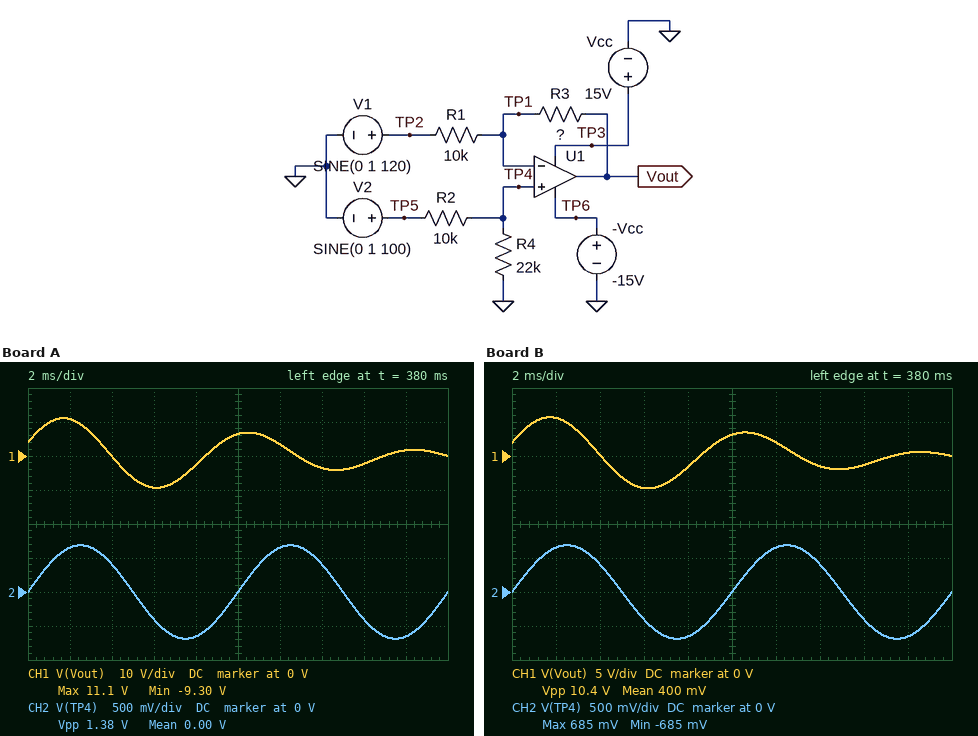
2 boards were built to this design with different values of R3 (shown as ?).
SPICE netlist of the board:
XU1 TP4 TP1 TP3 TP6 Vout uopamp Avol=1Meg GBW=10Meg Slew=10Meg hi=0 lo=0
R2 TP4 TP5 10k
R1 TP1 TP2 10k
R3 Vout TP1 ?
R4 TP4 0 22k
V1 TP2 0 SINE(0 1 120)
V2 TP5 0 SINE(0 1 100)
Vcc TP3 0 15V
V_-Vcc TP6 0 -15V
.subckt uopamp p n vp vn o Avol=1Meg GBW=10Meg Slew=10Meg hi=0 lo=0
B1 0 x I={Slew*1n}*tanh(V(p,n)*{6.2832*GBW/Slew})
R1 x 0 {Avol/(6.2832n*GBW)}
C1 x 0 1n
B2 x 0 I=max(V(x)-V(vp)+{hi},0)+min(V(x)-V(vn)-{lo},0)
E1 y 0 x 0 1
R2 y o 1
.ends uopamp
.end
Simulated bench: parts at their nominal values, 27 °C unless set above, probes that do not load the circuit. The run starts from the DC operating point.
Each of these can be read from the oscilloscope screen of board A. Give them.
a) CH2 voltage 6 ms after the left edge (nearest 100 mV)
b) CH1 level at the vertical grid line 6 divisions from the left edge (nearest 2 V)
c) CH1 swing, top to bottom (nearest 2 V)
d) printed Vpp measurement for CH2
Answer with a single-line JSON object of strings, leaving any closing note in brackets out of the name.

{"CH2 voltage 6 ms after the left edge": "-400 mV", "CH1 level at the vertical grid line 6 divisions from the left edge": "4 V", "CH1 swing, top to bottom": "20 V", "printed Vpp measurement for CH2": "1.38 V"}
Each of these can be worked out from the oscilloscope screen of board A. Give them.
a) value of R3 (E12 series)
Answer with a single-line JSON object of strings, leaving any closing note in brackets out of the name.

{"value of R3": "68 kΩ"}
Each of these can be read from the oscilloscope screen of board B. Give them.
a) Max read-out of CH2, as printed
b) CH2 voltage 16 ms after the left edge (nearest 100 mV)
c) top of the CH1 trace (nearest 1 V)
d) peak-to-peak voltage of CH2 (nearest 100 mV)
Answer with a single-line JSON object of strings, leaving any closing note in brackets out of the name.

{"Max read-out of CH2, as printed": "685 mV", "CH2 voltage 16 ms after the left edge": "-400 mV", "top of the CH1 trace": "6 V", "peak-to-peak voltage of CH2": "1.4 V"}
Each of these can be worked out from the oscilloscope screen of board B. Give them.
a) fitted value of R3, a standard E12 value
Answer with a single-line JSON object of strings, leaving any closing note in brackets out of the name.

{"fitted value of R3, a standard E12 value": "33 kΩ"}
